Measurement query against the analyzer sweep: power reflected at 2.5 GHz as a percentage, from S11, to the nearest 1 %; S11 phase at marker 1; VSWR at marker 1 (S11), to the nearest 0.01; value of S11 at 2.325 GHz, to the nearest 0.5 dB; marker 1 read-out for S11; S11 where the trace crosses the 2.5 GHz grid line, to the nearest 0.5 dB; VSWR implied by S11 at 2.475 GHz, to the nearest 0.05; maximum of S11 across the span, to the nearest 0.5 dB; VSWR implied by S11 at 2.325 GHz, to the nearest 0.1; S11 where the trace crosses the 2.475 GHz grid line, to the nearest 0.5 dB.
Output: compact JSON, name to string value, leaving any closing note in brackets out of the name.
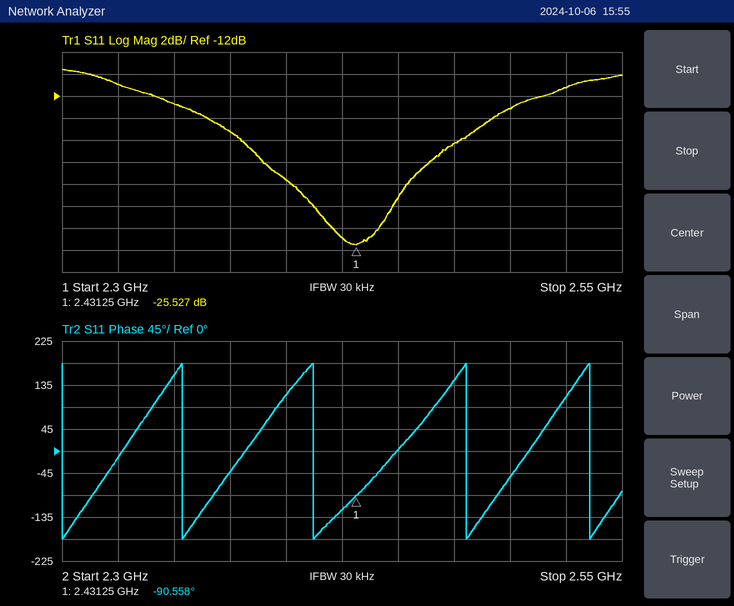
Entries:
{"power reflected at 2.5 GHz as a percentage, from S11, to the nearest 1 %": "5 %", "S11 phase at marker 1": "-90.558°", "VSWR at marker 1 (S11), to the nearest 0.01": "1.11", "value of S11 at 2.325 GHz, to the nearest 0.5 dB": "-11.0 dB", "marker 1 read-out for S11": "-25.527 dB", "S11 where the trace crosses the 2.5 GHz grid line, to the nearest 0.5 dB": "-13.0 dB", "VSWR implied by S11 at 2.475 GHz, to the nearest 0.05": "1.35", "maximum of S11 across the span, to the nearest 0.5 dB": "-9.5 dB", "VSWR implied by S11 at 2.325 GHz, to the nearest 0.1": "1.8", "S11 where the trace crosses the 2.475 GHz grid line, to the nearest 0.5 dB": "-16.5 dB"}
